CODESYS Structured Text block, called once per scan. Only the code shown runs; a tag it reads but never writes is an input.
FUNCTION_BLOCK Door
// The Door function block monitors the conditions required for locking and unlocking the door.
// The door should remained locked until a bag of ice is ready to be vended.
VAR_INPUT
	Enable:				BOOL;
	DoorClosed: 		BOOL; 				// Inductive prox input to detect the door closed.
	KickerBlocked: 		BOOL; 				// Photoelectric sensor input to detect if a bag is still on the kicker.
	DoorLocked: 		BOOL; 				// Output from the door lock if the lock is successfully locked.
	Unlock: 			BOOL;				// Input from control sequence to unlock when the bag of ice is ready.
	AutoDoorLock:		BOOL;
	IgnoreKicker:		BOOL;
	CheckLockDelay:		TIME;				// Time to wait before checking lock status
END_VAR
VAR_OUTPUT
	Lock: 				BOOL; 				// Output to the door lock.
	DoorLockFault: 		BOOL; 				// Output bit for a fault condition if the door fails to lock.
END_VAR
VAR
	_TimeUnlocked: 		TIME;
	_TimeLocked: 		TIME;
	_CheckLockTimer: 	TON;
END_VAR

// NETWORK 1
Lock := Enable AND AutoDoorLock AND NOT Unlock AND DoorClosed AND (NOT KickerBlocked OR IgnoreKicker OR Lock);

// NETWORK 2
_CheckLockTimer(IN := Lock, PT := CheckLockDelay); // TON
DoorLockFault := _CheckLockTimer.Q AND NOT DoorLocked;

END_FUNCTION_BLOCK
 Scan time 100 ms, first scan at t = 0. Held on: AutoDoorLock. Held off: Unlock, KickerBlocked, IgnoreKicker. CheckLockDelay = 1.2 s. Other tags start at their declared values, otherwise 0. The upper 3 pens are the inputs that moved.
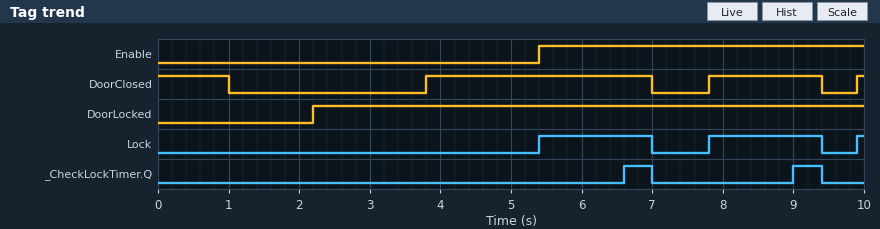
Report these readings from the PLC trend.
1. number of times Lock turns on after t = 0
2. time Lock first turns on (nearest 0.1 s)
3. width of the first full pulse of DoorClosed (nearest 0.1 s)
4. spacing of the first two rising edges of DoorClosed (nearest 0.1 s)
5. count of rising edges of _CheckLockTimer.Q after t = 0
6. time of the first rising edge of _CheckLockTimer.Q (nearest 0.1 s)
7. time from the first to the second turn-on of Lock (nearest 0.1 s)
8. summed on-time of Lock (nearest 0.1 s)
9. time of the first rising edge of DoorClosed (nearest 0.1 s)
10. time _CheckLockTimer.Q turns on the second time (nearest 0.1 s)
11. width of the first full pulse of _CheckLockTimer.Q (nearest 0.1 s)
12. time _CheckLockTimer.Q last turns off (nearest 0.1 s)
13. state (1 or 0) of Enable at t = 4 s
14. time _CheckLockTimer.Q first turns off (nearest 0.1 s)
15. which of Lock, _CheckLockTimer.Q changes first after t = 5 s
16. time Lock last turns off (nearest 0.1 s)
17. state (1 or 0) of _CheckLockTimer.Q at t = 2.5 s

3
5.4 s
3.2 s
4.0 s
2
6.6 s
2.4 s
3.3 s
3.8 s
9.0 s
0.4 s
9.4 s
0
7.0 s
Lock
9.4 s
0
